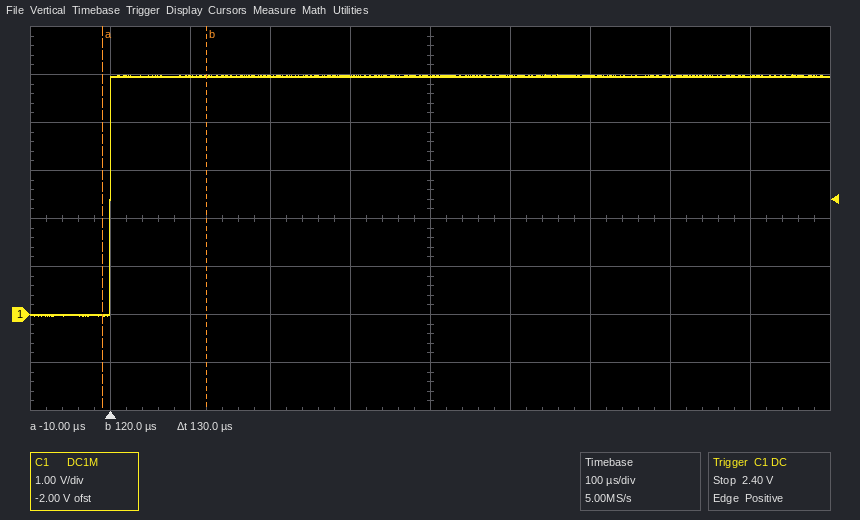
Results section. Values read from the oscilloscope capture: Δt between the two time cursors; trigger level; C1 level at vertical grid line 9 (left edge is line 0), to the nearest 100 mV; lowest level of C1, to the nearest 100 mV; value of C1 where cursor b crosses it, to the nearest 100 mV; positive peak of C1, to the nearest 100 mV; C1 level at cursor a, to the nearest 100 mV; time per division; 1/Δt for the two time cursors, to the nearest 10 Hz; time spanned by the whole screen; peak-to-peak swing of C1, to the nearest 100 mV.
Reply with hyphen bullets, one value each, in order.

- 130 µs
- 2.40 V
- 5.0 V
- 0.0 V
- 5.0 V
- 5.0 V
- 0.0 V
- 100 µs
- 7.69 kHz
- 1 ms
- 5.0 V
